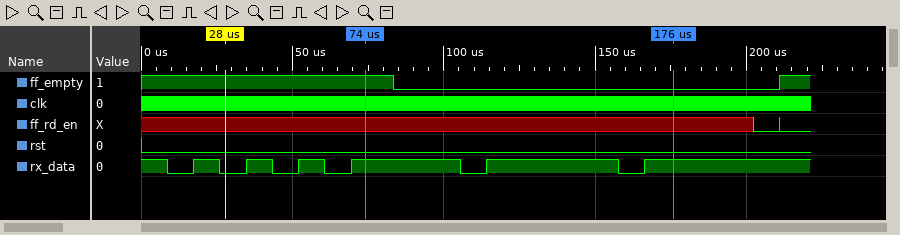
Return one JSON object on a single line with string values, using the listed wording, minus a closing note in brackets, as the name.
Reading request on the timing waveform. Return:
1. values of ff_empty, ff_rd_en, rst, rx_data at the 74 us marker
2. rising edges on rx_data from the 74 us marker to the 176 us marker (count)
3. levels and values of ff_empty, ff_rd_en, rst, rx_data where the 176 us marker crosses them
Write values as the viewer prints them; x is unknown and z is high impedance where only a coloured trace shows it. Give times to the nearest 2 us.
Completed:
{"values of ff_empty, ff_rd_en, rst, rx_data at the 74 us marker": "ff_empty=1, ff_rd_en=x, rst=0, rx_data=1", "rising edges on rx_data from the 74 us marker to the 176 us marker": "2", "levels and values of ff_empty, ff_rd_en, rst, rx_data where the 176 us marker crosses them": "ff_empty=0, ff_rd_en=x, rst=0, rx_data=1"}
